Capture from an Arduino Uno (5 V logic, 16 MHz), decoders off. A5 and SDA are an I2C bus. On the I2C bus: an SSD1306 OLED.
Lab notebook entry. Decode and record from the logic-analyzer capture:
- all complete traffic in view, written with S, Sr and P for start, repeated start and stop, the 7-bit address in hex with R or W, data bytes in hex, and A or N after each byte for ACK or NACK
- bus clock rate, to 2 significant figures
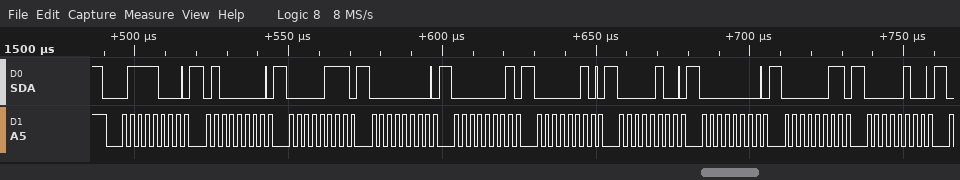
S 3CW A 40 A 07 A 00 A 01 A 02 A 04 A 00 A 03 A 04 A
400 kHz
